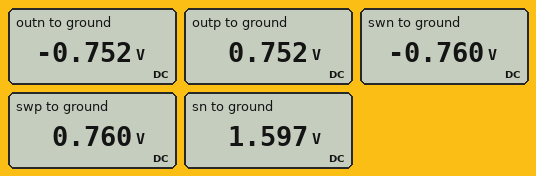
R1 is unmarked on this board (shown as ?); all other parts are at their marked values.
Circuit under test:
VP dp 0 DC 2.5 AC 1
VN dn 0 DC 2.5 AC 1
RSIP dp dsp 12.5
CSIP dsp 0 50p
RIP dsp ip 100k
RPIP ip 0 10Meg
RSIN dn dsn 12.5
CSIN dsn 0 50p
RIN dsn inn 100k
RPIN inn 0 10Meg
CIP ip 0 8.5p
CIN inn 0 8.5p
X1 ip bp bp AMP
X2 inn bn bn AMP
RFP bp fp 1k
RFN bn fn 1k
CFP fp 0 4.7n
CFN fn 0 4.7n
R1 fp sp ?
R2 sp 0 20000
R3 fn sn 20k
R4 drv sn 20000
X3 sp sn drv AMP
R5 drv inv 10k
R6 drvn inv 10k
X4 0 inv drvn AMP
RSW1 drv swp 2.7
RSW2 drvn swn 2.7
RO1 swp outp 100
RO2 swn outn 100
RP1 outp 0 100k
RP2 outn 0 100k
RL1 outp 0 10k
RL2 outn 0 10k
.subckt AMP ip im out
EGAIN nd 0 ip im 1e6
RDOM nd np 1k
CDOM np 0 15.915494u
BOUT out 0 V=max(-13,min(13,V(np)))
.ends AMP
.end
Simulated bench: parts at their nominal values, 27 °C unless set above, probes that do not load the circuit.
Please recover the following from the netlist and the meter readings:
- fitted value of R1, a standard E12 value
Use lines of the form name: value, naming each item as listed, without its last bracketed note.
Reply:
fitted value of R1, a standard E12 value: 10 kΩ
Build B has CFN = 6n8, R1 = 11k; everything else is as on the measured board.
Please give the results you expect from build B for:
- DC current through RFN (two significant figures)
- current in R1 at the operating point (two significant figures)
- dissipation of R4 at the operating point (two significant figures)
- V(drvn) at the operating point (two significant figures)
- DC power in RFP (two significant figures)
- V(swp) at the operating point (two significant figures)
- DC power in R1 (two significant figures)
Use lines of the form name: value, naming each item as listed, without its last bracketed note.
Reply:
DC current through RFN: 44 µA
current in R1 at the operating point: 77 µA
dissipation of R4 at the operating point: 39 µW
V(drvn) at the operating point: -660 mV
DC power in RFP: 6.0 µW
V(swp) at the operating point: 660 mV
DC power in R1: 66 µW
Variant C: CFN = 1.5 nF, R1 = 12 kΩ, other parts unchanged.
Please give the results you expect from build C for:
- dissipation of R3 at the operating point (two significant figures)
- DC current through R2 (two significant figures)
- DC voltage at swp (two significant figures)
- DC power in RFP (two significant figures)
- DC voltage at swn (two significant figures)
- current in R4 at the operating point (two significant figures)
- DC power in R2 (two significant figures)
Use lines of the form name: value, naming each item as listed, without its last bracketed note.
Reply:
dissipation of R3 at the operating point: 43 µW
DC current through R2: 75 µA
DC voltage at swp: 570 mV
DC power in RFP: 5.6 µW
DC voltage at swn: -570 mV
current in R4 at the operating point: 46 µA
DC power in R2: 110 µW
